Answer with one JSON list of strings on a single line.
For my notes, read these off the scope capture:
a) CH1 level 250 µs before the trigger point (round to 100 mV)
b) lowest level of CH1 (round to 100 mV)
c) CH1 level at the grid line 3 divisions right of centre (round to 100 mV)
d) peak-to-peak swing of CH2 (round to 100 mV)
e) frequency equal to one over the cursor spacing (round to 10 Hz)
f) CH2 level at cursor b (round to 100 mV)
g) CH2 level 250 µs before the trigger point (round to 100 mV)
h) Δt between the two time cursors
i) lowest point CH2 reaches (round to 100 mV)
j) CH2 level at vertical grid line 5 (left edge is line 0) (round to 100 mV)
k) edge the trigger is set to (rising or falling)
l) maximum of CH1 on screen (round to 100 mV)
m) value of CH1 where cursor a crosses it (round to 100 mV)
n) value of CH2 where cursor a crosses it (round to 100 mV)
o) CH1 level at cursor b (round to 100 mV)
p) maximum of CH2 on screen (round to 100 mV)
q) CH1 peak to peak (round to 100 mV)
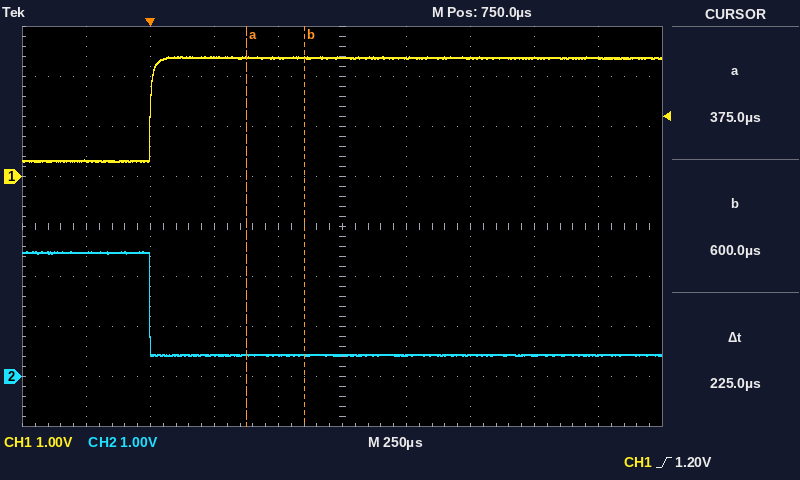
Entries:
["300 mV", "300 mV", "2.4 V", "2.1 V", "4.44 kHz", "400 mV", "2.5 V", "225 µs", "400 mV", "400 mV", "rising", "2.4 V", "2.4 V", "400 mV", "2.4 V", "2.5 V", "2.1 V"]
